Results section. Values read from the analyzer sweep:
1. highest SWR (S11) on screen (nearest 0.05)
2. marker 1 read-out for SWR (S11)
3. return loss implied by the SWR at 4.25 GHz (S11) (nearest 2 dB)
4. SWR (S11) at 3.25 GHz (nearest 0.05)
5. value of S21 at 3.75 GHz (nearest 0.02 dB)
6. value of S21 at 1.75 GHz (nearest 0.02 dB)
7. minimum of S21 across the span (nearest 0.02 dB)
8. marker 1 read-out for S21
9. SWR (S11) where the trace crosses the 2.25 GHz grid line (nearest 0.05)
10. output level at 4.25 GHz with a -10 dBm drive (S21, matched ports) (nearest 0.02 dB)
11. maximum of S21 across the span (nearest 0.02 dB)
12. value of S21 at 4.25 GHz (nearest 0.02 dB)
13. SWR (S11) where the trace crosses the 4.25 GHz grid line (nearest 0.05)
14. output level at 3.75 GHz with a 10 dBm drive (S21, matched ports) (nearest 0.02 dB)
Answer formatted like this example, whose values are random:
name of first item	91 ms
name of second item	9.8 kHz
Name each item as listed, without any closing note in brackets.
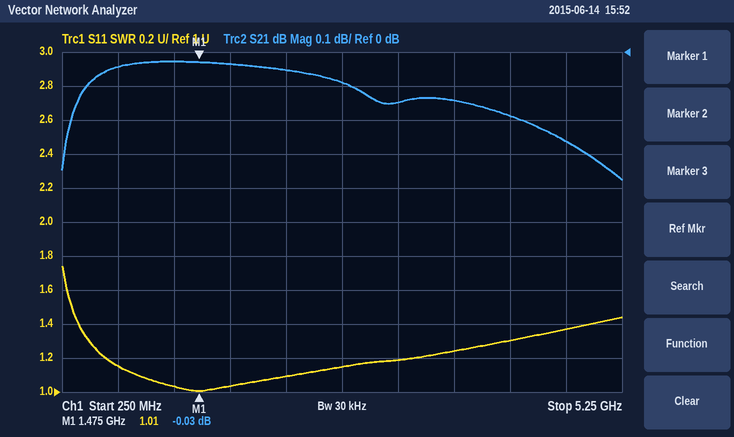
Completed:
highest SWR (S11) on screen	1.75
marker 1 read-out for SWR	1.01
return loss implied by the SWR at 4.25 GHz (S11)	18 dB
SWR (S11) at 3.25 GHz	1.20
value of S21 at 3.75 GHz	-0.14 dB
value of S21 at 1.75 GHz	-0.04 dB
minimum of S21 across the span	-0.38 dB
marker 1 read-out for S21	-0.03 dB
SWR (S11) where the trace crosses the 2.25 GHz grid line	1.10
output level at 4.25 GHz with a -10 dBm drive (S21, matched ports)	-10.18 dBm
maximum of S21 across the span	-0.02 dB
value of S21 at 4.25 GHz	-0.18 dB
SWR (S11) where the trace crosses the 4.25 GHz grid line	1.30
output level at 3.75 GHz with a 10 dBm drive (S21, matched ports)	9.86 dBm
